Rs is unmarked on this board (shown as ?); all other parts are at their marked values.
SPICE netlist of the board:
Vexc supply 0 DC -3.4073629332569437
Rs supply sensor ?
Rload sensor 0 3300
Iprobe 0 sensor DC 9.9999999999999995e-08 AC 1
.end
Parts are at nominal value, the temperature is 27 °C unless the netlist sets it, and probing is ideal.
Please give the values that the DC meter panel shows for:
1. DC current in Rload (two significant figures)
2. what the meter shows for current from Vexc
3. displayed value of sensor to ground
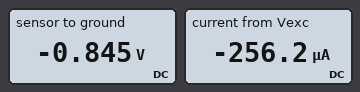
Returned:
260 µA
-256.2 µA
-0.845 V
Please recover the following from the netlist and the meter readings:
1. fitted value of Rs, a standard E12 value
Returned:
10 kΩ
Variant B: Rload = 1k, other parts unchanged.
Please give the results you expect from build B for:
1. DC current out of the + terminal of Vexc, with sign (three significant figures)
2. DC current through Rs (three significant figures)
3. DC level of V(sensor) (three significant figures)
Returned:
-310 µA
310 µA
-310 mV
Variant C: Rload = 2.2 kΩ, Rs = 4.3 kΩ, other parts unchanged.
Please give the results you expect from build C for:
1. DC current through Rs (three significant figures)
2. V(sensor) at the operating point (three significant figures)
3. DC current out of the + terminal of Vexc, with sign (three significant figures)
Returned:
524 µA
-1.15 V
-524 µA
